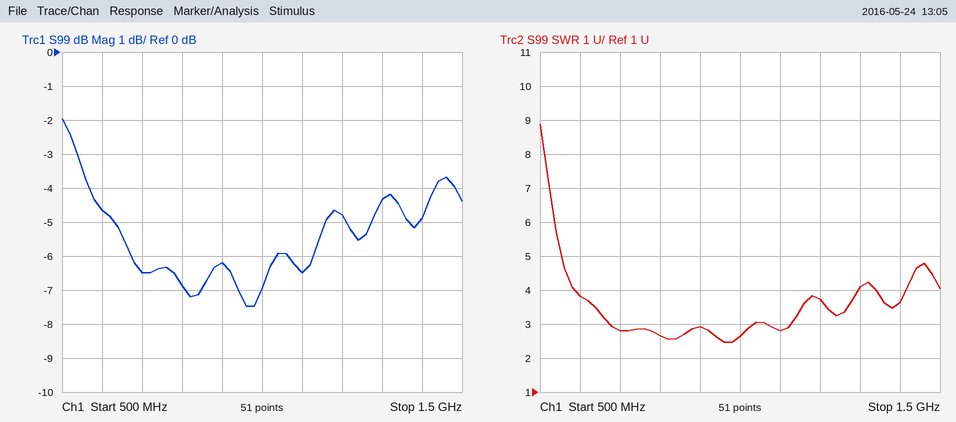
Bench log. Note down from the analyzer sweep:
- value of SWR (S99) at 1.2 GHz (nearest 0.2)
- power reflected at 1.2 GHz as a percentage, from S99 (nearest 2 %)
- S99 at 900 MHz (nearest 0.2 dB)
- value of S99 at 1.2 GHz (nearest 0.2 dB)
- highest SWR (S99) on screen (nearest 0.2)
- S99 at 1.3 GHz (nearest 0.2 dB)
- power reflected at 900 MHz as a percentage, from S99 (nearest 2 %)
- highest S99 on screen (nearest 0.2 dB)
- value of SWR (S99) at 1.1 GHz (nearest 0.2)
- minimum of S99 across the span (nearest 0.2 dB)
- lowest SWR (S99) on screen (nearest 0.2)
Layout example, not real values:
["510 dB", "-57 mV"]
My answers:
["3.8", "34 %", "-6.2 dB", "-4.8 dB", "8.8", "-4.4 dB", "24 %", "-2.0 dB", "2.8", "-7.4 dB", "2.4"]
